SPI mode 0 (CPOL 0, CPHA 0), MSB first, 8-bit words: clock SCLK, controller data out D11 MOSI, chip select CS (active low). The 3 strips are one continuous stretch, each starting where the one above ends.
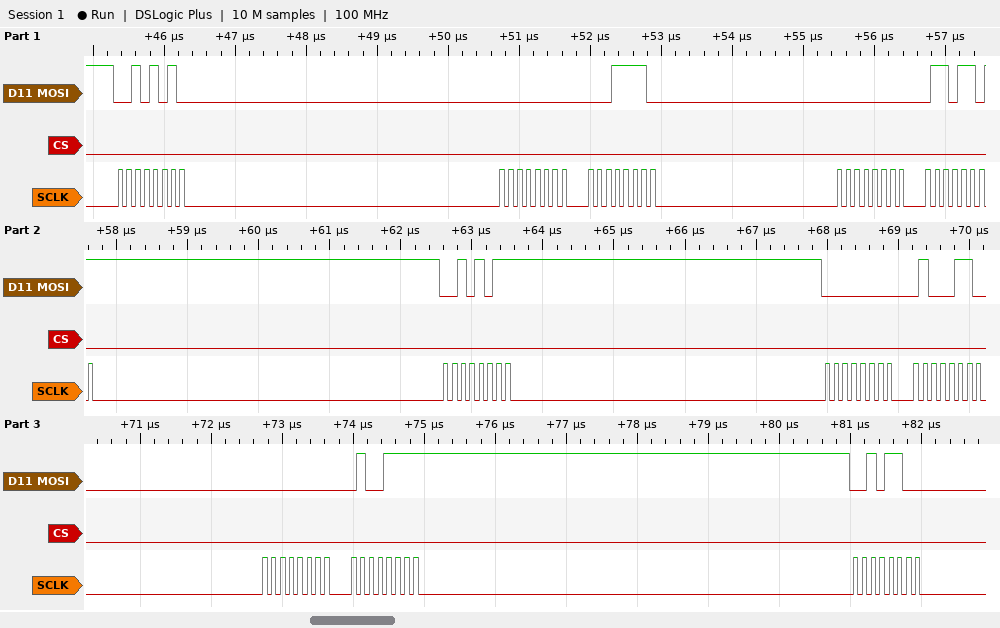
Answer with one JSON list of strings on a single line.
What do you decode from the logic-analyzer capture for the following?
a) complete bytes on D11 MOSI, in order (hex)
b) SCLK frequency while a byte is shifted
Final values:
["2A 00 1E 00 6D 2B 00 46 00 4F 2C", "8 MHz"]
